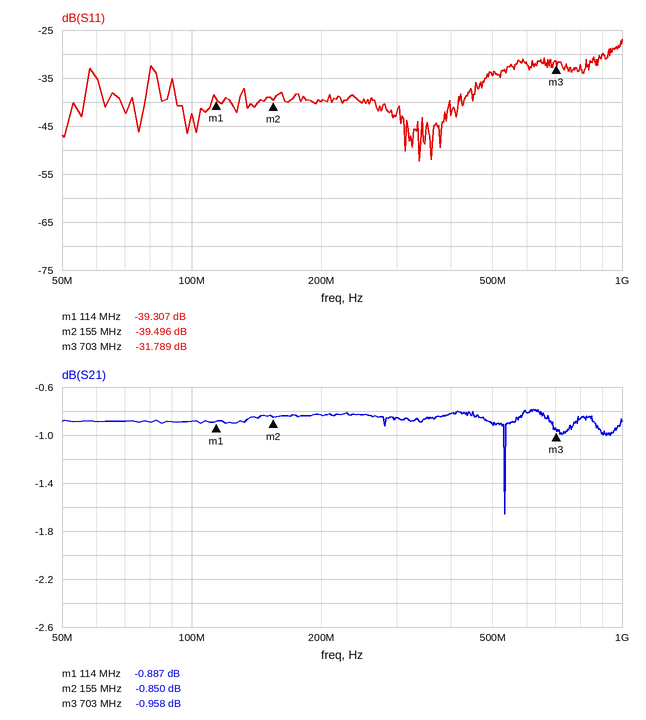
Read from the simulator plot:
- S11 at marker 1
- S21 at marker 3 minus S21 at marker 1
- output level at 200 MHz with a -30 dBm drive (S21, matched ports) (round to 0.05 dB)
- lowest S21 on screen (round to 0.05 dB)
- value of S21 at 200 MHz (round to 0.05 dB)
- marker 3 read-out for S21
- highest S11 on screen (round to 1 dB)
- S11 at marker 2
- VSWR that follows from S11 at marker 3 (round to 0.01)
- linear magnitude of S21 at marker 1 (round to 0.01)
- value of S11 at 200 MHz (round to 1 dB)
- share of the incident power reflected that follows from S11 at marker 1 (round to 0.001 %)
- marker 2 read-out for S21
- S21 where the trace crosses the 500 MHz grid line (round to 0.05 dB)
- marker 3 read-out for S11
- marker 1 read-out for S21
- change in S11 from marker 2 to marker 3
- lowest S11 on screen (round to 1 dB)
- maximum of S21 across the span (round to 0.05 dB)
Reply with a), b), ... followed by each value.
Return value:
a) -39.307 dB
b) -0.071 dB
c) -30.85 dBm
d) -1.65 dB
e) -0.85 dB
f) -0.958 dB
g) -27 dB
h) -39.496 dB
i) 1.05
j) 0.90
k) -40 dB
l) 0.012 %
m) -0.850 dB
n) -0.90 dB
o) -31.789 dB
p) -0.887 dB
q) 7.707 dB
r) -52 dB
s) -0.80 dB
